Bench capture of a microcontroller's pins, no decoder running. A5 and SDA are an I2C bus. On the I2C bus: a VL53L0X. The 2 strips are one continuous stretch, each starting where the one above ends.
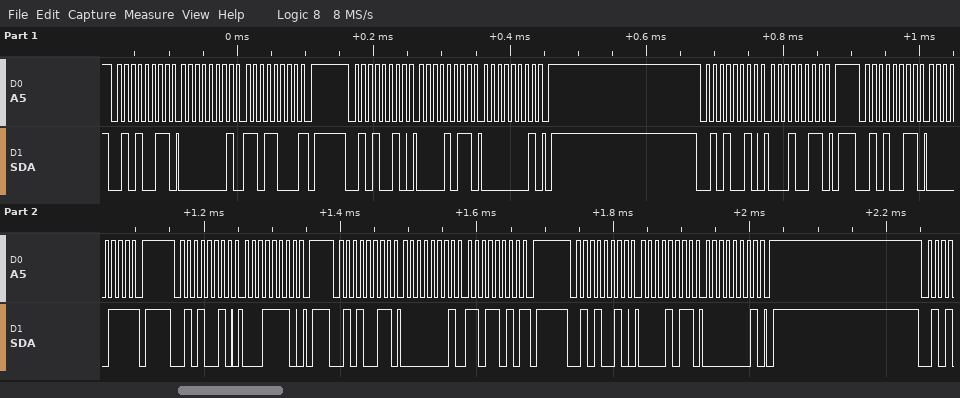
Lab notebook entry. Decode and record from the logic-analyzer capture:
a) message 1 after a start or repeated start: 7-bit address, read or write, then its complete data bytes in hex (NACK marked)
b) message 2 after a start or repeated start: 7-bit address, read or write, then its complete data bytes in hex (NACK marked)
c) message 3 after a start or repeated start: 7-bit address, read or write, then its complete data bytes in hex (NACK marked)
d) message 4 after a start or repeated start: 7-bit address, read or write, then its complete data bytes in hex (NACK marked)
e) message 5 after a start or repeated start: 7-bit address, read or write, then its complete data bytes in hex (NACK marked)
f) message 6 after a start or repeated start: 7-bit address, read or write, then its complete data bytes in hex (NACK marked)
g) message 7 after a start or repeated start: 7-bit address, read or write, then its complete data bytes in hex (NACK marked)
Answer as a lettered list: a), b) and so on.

a) 0x29 read: 01 D8 NACK
b) 0x29 write: 0B 01
c) 0x29 write: 13
d) 0x29 read: 07 NACK
e) 0x29 write: 1E
f) 0x29 read: 01 DA NACK
g) 0x29 write: 0B 01
